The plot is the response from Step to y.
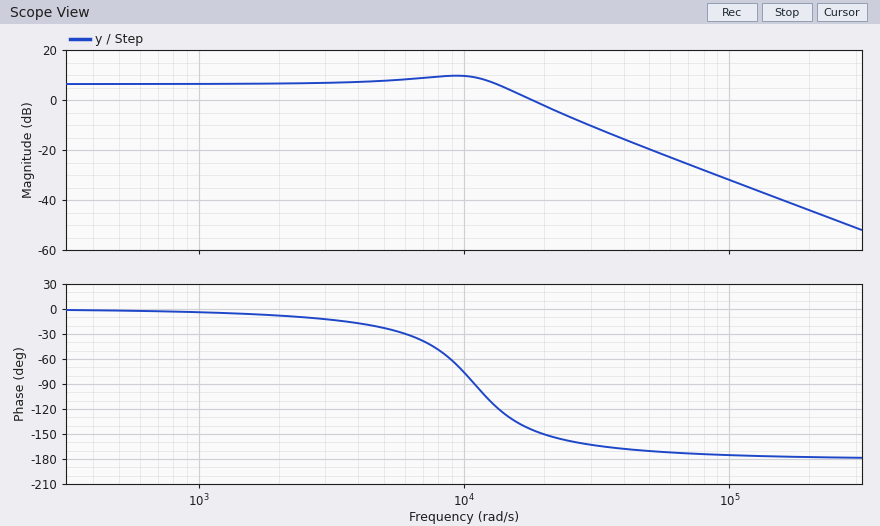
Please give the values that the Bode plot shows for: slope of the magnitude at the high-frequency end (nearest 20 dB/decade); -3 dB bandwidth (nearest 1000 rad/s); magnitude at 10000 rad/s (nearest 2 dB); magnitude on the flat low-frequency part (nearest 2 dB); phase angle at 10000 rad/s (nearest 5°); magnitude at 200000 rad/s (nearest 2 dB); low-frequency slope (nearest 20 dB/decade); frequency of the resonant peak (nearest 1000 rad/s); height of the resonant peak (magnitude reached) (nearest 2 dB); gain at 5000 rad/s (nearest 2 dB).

-40 dB/decade
15000 rad/s
10 dB
6 dB
-75°
-44 dB
0 dB/decade
9000 rad/s
10 dB
8 dB
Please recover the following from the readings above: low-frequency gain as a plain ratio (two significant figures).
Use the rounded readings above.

2.0
